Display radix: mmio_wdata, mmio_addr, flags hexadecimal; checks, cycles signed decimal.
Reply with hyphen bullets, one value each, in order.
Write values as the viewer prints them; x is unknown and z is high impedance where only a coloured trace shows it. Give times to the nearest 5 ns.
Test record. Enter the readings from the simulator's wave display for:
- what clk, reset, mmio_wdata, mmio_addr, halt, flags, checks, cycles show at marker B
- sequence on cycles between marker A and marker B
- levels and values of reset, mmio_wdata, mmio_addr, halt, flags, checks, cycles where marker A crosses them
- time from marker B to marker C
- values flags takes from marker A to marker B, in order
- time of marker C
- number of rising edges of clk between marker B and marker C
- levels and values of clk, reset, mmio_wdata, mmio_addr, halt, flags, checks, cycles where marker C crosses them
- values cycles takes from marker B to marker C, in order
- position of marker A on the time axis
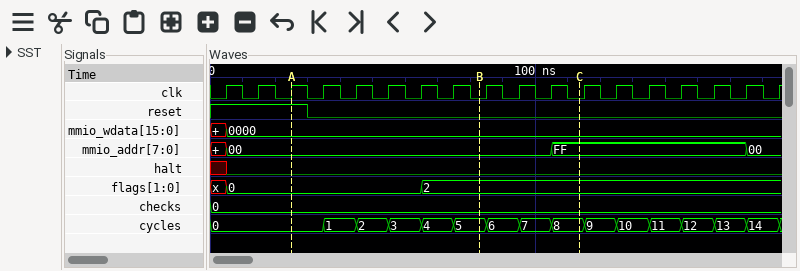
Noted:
- clk=0, reset=0, mmio_wdata=0000, mmio_addr=00, halt=0, flags=2, checks=0, cycles=5
- 0, 1, 2, 3, 4, 5
- reset=1, mmio_wdata=0000, mmio_addr=00, halt=0, flags=0, checks=0, cycles=0
- 30 ns
- 0, 2
- 115 ns
- 3
- clk=0, reset=0, mmio_wdata=0000, mmio_addr=FF, halt=0, flags=2, checks=0, cycles=8
- 5, 6, 7, 8
- 25 ns
